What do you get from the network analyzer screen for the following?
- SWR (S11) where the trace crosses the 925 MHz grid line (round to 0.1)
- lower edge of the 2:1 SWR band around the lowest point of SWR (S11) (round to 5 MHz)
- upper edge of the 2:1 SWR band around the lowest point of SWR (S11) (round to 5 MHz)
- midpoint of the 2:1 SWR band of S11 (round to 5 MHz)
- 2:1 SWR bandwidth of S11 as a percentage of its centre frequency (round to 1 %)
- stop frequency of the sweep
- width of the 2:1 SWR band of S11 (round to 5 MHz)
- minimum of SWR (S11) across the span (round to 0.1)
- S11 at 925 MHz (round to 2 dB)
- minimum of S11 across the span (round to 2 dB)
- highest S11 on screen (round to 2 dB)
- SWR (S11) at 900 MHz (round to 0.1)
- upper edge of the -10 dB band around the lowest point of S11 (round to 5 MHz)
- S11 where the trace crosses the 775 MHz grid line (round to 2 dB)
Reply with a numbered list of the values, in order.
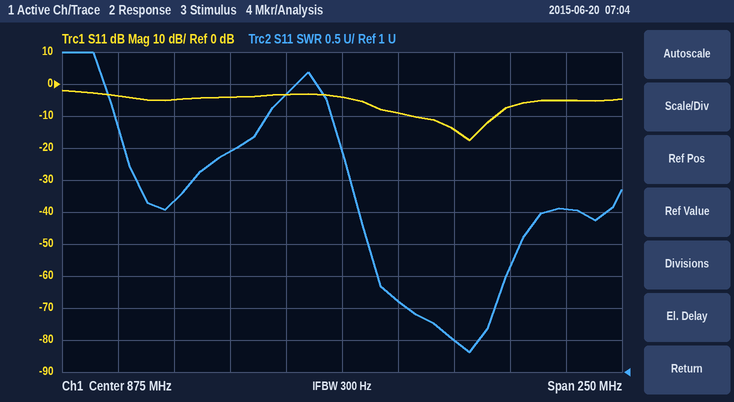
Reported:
1. 1.5
2. 905 MHz
3. 945 MHz
4. 925 MHz
5. 4 %
6. 1 GHz
7. 40 MHz
8. 1.3
9. -14 dB
10. -18 dB
11. -2 dB
12. 2.1
13. 945 MHz
14. -4 dB
